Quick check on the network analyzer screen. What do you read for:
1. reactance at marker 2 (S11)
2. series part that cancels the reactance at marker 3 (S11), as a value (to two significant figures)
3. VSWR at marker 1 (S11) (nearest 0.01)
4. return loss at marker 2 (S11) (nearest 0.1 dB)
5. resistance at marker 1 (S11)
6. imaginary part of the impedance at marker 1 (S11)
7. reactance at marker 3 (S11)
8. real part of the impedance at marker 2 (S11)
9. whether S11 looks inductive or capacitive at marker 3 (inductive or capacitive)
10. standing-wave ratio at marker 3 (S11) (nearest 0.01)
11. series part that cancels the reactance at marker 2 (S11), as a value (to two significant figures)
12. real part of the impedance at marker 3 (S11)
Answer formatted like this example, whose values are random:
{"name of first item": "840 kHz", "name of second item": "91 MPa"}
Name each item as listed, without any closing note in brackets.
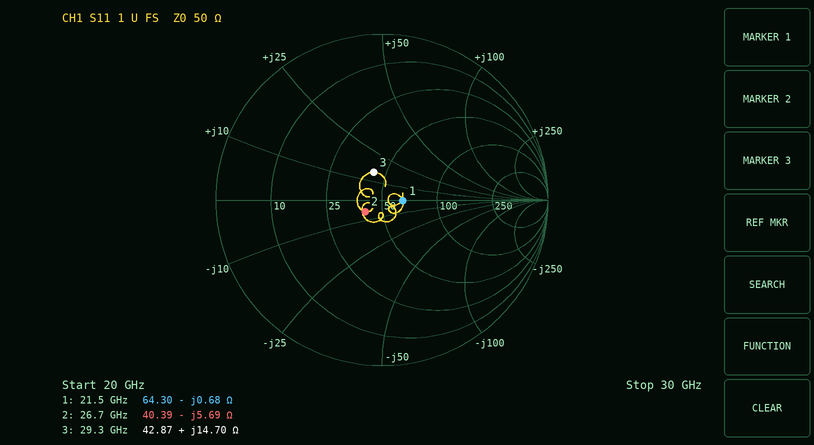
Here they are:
{"reactance at marker 2": "-5.69 Ω", "series part that cancels the reactance at marker 3 (S11), as a value": "370 fF", "VSWR at marker 1 (S11)": "1.29", "return loss at marker 2 (S11)": "18.2 dB", "resistance at marker 1": "64.30 Ω", "imaginary part of the impedance at marker 1": "-0.68 Ω", "reactance at marker 3": "+14.70 Ω", "real part of the impedance at marker 2": "40.39 Ω", "whether S11 looks inductive or capacitive at marker 3": "inductive", "standing-wave ratio at marker 3 (S11)": "1.42", "series part that cancels the reactance at marker 2 (S11), as a value": "34 pH", "real part of the impedance at marker 3": "42.87 Ω"}
